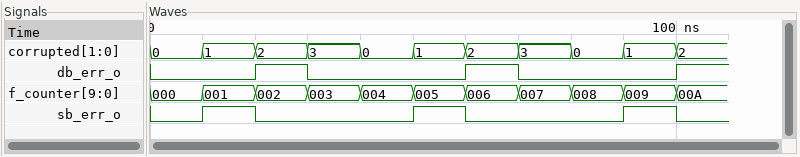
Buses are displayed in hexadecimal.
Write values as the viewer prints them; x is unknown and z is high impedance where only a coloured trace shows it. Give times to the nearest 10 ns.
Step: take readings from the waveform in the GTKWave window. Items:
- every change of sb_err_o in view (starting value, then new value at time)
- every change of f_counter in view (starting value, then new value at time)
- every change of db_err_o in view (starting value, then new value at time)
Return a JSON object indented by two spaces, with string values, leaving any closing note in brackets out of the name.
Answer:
{
  "every change of sb_err_o in view": "0, 1 at 10 ns, 0 at 20 ns, 1 at 50 ns, 0 at 60 ns, 1 at 90 ns, 0 at 100 ns",
  "every change of f_counter in view": "000, 001 at 10 ns, 002 at 20 ns, 003 at 30 ns, 004 at 40 ns, 005 at 50 ns, 006 at 60 ns, 007 at 70 ns, 008 at 80 ns, 009 at 90 ns, 00A at 100 ns",
  "every change of db_err_o in view": "0, 1 at 20 ns, 0 at 30 ns, 1 at 60 ns, 0 at 70 ns, 1 at 100 ns"
}
